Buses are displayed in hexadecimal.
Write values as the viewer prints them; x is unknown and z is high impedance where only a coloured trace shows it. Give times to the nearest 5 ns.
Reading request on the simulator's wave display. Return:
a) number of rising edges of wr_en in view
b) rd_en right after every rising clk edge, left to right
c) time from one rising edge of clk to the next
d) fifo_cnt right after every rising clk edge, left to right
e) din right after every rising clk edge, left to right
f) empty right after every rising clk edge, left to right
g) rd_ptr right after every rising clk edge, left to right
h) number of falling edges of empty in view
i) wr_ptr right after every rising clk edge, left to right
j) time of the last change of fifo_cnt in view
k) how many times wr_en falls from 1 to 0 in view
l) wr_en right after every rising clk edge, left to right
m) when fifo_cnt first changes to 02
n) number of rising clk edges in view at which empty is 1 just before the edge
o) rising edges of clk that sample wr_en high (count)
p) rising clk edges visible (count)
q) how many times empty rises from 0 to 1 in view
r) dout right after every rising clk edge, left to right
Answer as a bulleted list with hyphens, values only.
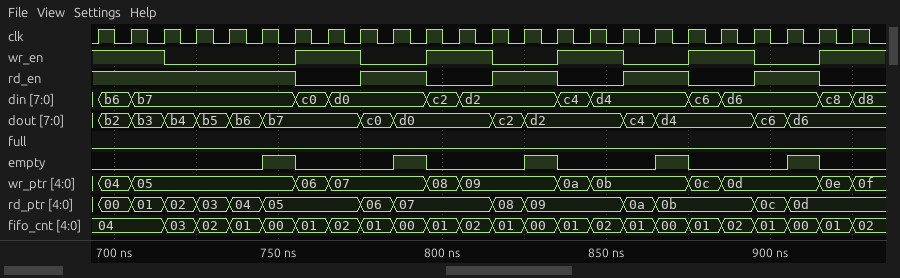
- 5
- 1 1 1 1 1 1 0 0 1 1 0 0 1 1 0 0 1 1 0 0 1 1 0 0
- 10 ns
- 04, 04, 03, 02, 01, 00, 01, 02, 01, 00, 01, 02, 01, 00, 01, 02, 01, 00, 01, 02, 01, 00, 01, 02
- b6, b7, b7, b7, b7, b7, c0, d0, d0, d0, c2, d2, d2, d2, c4, d4, d4, d4, c6, d6, d6, d6, c8, d8
- 0 0 0 0 0 1 0 0 0 1 0 0 0 1 0 0 0 1 0 0 0 1 0 0
- 00, 01, 02, 03, 04, 05, 05, 05, 06, 07, 07, 07, 08, 09, 09, 09, 0a, 0b, 0b, 0b, 0c, 0d, 0d, 0d
- 5
- 04, 05, 05, 05, 05, 05, 06, 07, 07, 07, 08, 09, 09, 09, 0a, 0b, 0b, 0b, 0c, 0d, 0d, 0d, 0e, 0f
- 925 ns
- 5
- 1 1 0 0 0 0 1 1 0 0 1 1 0 0 1 1 0 0 1 1 0 0 1 1
- 725 ns
- 5
- 12
- 24
- 5
- b2, b3, b4, b5, b6, b7, b7, b7, c0, d0, d0, d0, c2, d2, d2, d2, c4, d4, d4, d4, c6, d6, d6, d6
